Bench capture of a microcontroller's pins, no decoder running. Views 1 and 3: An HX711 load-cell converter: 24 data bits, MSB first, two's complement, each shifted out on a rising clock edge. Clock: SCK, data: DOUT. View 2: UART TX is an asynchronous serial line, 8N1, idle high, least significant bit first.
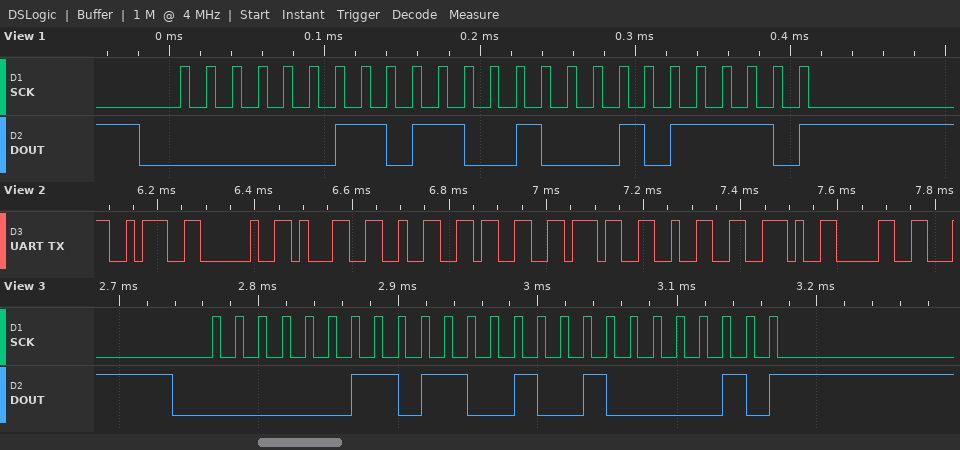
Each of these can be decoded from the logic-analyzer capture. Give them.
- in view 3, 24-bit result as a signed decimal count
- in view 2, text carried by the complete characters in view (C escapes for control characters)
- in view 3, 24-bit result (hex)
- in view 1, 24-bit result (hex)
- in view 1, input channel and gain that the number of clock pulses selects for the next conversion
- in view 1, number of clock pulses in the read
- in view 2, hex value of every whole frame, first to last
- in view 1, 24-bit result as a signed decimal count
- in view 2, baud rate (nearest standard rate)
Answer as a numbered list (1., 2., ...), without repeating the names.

1. 222338
2. ": 12372.0"
3. 0x036482
4. 0x03645E
5. channel A, gain 128
6. 25
7. 3A 20 31 32 33 37 32 2E 30
8. 222302
9. 57600 baud
